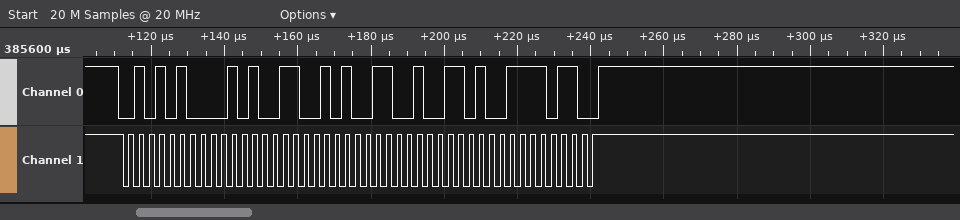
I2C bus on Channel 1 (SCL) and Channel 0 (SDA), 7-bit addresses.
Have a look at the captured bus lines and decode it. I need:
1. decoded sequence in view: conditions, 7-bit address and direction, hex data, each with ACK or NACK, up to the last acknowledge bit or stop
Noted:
start, address 2A write ACK, 53 ACK, 53 ACK, 4D ACK, 7B ACK, stop
